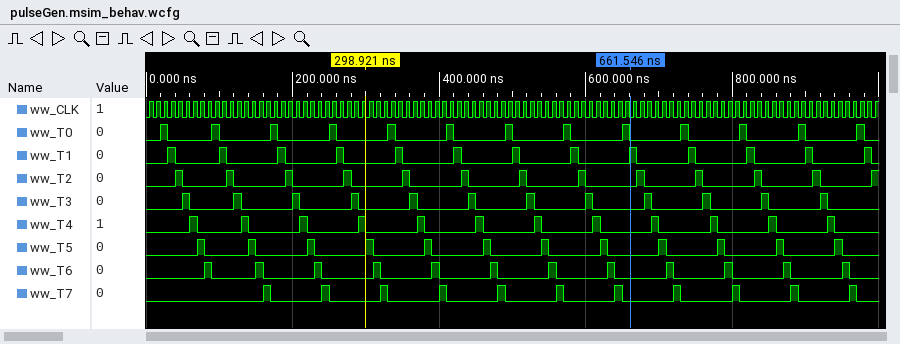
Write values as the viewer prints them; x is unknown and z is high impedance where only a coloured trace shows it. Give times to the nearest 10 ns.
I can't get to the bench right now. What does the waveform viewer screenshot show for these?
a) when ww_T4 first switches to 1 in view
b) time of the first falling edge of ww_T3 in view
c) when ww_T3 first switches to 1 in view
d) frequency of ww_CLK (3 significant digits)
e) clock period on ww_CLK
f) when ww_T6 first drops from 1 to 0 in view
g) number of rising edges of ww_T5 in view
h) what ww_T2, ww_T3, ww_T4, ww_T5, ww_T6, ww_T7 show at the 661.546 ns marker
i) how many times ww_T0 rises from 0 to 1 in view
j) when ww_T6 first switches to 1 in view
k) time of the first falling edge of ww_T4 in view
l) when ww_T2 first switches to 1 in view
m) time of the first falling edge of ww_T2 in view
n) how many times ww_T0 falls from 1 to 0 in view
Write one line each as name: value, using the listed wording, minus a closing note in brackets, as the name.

when ww_T4 first switches to 1 in view: 60 ns
time of the first falling edge of ww_T3 in view: 60 ns
when ww_T3 first switches to 1 in view: 50 ns
frequency of ww_CLK: 100 MHz
clock period on ww_CLK: 10 ns
when ww_T6 first drops from 1 to 0 in view: 90 ns
number of rising edges of ww_T5 in view: 12
what ww_T2, ww_T3, ww_T4, ww_T5, ww_T6, ww_T7 show at the 661.546 ns marker: ww_T2=0, ww_T3=0, ww_T4=0, ww_T5=0, ww_T6=0, ww_T7=0
how many times ww_T0 rises from 0 to 1 in view: 13
when ww_T6 first switches to 1 in view: 80 ns
time of the first falling edge of ww_T4 in view: 70 ns
when ww_T2 first switches to 1 in view: 40 ns
time of the first falling edge of ww_T2 in view: 50 ns
how many times ww_T0 falls from 1 to 0 in view: 13
